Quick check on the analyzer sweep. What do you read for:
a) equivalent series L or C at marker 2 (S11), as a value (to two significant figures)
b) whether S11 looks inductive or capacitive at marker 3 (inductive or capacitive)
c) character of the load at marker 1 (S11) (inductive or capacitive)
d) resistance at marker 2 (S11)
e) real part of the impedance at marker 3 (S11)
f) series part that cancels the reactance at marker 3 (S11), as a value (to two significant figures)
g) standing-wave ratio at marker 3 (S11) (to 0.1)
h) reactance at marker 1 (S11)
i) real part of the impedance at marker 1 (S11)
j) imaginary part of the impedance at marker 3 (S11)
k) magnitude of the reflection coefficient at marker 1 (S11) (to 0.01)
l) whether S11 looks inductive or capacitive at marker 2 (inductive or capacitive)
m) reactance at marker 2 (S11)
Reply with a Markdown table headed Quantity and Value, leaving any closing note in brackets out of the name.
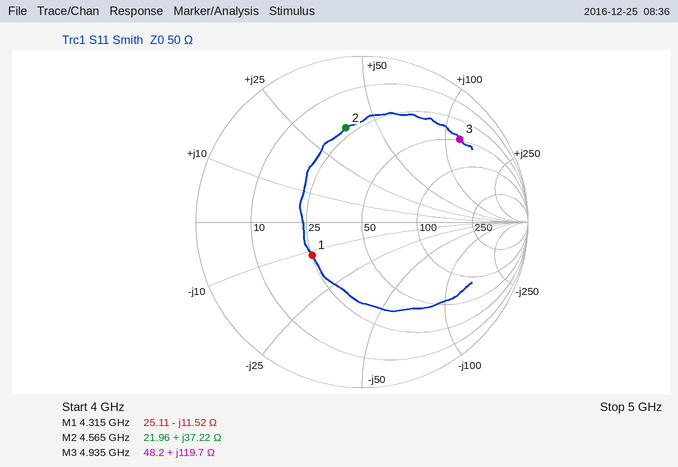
| Quantity | Value |
|---|---|
| equivalent series L or C at marker 2 (S11), as a value | 1.3 nH |
| whether S11 looks inductive or capacitive at marker 3 | inductive |
| character of the load at marker 1 (S11) | capacitive |
| resistance at marker 2 | 21.96 Ω |
| real part of the impedance at marker 3 | 48.2 Ω |
| series part that cancels the reactance at marker 3 (S11), as a value | 270 fF |
| standing-wave ratio at marker 3 (S11) | 7.8 |
| reactance at marker 1 | -11.52 Ω |
| real part of the impedance at marker 1 | 25.11 Ω |
| imaginary part of the impedance at marker 3 | +119.7 Ω |
| magnitude of the reflection coefficient at marker 1 (S11) | 0.36 |
| whether S11 looks inductive or capacitive at marker 2 | inductive |
| reactance at marker 2 | +37.22 Ω |
